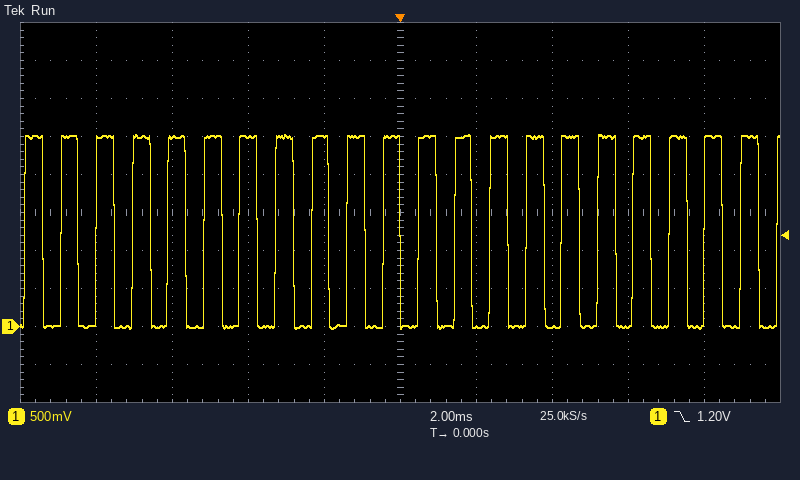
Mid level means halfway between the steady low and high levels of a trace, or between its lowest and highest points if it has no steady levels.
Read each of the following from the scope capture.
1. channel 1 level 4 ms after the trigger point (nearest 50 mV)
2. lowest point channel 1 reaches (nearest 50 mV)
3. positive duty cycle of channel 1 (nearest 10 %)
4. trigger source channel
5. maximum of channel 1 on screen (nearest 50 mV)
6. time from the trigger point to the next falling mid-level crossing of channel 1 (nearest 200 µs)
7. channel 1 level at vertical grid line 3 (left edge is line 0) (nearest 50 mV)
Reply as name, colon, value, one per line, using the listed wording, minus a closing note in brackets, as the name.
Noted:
channel 1 level 4 ms after the trigger point: 0 mV
lowest point channel 1 reaches: -50 mV
positive duty cycle of channel 1: 50 %
trigger source channel: channel 1
maximum of channel 1 on screen: 2.55 V
time from the trigger point to the next falling mid-level crossing of channel 1: 1.0 ms
channel 1 level at vertical grid line 3 (left edge is line 0): 2.50 V
